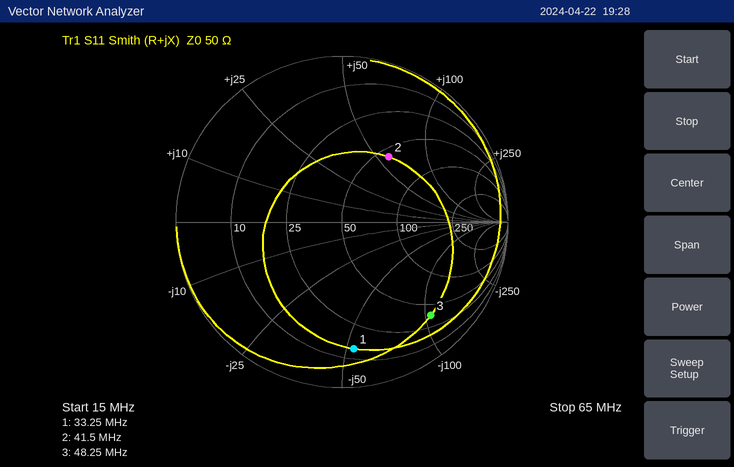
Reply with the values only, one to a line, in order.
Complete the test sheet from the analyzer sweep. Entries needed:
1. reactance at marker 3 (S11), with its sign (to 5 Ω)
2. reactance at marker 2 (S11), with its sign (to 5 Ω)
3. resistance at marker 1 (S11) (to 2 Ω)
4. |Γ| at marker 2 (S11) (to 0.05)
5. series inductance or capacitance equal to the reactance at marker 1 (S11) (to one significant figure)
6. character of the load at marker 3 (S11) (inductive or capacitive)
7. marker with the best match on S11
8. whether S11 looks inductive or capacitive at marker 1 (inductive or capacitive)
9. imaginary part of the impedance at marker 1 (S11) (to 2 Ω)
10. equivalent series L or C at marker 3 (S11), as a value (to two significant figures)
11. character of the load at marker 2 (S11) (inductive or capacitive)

-105 Ω
+60 Ω
14 Ω
0.50
90 pF
capacitive
marker 2
capacitive
-52 Ω
31 pF
inductive
